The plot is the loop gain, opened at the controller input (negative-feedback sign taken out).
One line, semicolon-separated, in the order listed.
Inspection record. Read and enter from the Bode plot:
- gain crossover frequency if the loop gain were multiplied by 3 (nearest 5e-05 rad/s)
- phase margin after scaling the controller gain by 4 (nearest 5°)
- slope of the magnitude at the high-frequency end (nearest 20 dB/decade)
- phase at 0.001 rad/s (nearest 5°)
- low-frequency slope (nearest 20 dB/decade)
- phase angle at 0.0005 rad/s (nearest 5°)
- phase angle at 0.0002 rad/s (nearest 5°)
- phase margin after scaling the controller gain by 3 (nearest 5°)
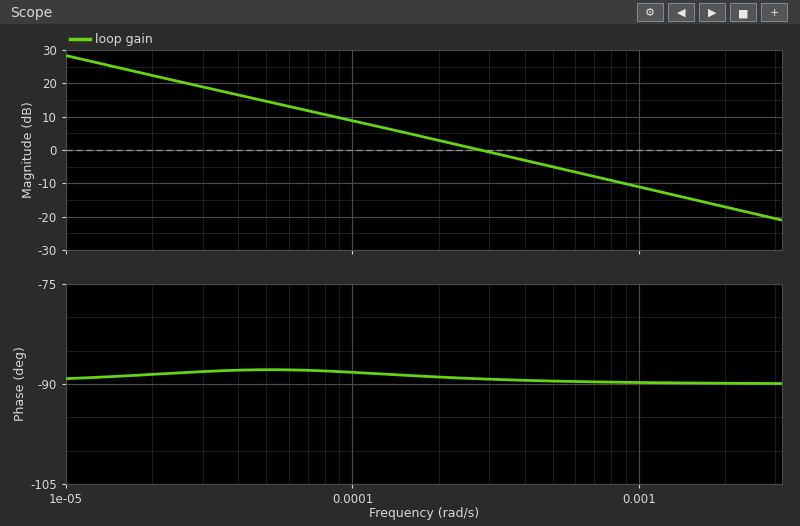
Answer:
0.00085 rad/s; 90°; -20 dB/decade; -90°; -20 dB/decade; -90°; -90°; 90°
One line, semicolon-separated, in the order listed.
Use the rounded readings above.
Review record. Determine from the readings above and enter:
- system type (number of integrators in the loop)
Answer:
1
